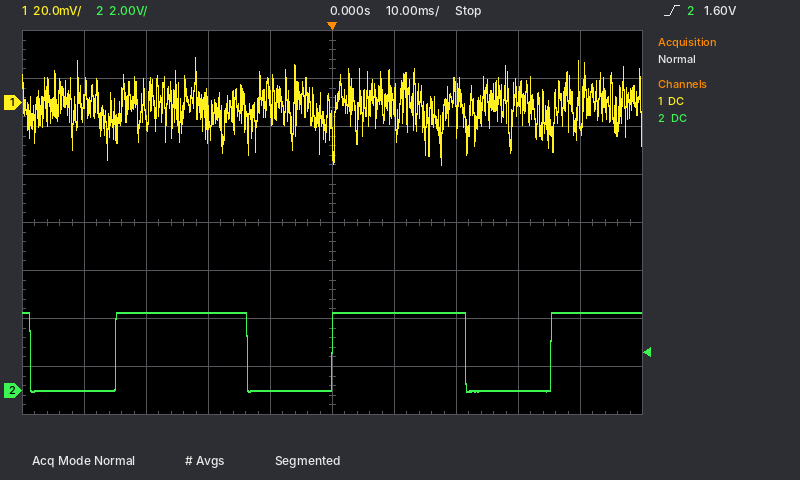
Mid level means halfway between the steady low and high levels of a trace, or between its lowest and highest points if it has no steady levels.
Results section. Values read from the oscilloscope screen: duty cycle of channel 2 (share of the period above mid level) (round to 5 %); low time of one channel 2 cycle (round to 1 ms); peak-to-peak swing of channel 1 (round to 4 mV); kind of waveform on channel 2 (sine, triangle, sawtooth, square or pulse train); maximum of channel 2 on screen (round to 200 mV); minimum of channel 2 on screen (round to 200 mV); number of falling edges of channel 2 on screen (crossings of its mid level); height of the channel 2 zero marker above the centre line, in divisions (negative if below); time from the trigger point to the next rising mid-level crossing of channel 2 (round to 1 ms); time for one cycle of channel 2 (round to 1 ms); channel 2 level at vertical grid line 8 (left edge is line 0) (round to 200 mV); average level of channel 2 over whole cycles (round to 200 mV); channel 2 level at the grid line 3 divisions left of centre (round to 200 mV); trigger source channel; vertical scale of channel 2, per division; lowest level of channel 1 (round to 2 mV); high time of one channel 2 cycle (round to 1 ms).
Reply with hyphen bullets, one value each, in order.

- 60 %
- 14 ms
- 44 mV
- pulse train
- 3.2 V
- 0.0 V
- 3
- -3.5 div
- 35 ms
- 35 ms
- 0.0 V
- 2.0 V
- 3.2 V
- channel 2
- 2 V
- -26 mV
- 21 ms
